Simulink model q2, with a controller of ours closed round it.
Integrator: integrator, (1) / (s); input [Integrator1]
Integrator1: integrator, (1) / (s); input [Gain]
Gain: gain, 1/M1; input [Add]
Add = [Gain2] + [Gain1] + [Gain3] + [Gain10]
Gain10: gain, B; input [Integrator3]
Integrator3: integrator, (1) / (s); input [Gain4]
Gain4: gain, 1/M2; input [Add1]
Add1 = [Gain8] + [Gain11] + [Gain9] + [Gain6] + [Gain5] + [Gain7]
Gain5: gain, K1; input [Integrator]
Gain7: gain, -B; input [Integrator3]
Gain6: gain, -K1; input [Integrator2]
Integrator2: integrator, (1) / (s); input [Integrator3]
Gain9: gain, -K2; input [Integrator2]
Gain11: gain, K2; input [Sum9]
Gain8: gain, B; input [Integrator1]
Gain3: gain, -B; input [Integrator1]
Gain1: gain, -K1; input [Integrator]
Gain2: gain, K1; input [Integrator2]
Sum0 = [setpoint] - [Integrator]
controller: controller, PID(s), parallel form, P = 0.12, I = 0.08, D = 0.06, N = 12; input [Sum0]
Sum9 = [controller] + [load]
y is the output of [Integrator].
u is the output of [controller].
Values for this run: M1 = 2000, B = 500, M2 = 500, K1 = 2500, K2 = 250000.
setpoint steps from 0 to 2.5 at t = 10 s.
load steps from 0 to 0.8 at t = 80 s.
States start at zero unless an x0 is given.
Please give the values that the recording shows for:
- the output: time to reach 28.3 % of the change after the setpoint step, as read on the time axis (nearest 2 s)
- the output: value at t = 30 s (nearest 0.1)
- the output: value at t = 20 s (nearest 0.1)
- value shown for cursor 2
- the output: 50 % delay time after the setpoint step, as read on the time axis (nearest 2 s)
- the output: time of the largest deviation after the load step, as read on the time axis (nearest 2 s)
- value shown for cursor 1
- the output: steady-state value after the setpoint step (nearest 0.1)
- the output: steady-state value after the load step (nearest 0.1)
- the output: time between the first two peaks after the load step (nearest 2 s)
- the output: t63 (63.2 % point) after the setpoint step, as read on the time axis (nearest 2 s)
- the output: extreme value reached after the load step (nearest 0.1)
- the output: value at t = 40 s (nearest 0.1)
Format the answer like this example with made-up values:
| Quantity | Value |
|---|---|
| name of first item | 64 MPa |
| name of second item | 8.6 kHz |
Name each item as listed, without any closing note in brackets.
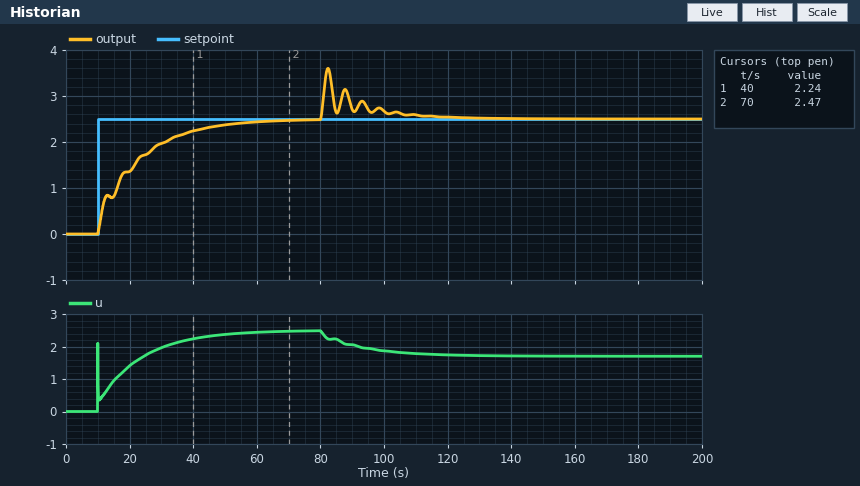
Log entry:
| Quantity | Value |
|---|---|
| the output: time to reach 28.3 % of the change after the setpoint step, as read on the time axis | 12 s |
| the output: value at t = 30 s | 2.0 |
| the output: value at t = 20 s | 1.4 |
| value shown for cursor 2 | 2.47 |
| the output: 50 % delay time after the setpoint step, as read on the time axis | 18 s |
| the output: time of the largest deviation after the load step, as read on the time axis | 82 s |
| value shown for cursor 1 | 2.24 |
| the output: steady-state value after the setpoint step | 2.5 |
| the output: steady-state value after the load step | 2.5 |
| the output: time between the first two peaks after the load step | 6 s |
| the output: t63 (63.2 % point) after the setpoint step, as read on the time axis | 22 s |
| the output: extreme value reached after the load step | 3.6 |
| the output: value at t = 40 s | 2.2 |
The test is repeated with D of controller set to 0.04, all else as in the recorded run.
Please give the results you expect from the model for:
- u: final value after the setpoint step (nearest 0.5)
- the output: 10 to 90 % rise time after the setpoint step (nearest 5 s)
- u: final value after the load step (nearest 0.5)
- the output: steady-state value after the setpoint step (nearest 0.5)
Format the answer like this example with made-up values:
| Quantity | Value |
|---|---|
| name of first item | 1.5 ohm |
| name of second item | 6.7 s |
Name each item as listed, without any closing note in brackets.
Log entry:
| Quantity | Value |
|---|---|
| u: final value after the setpoint step | 2.5 |
| the output: 10 to 90 % rise time after the setpoint step | 30 s |
| u: final value after the load step | 1.5 |
| the output: steady-state value after the setpoint step | 2.5 |
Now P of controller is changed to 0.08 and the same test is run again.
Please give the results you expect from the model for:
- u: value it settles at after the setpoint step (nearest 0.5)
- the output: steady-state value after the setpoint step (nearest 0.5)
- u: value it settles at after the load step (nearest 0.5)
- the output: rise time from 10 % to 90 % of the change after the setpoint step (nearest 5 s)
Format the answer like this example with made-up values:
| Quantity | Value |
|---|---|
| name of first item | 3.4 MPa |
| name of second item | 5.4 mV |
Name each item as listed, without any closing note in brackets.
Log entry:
| Quantity | Value |
|---|---|
| u: value it settles at after the setpoint step | 2.5 |
| the output: steady-state value after the setpoint step | 2.5 |
| u: value it settles at after the load step | 1.5 |
| the output: rise time from 10 % to 90 % of the change after the setpoint step | 30 s |
